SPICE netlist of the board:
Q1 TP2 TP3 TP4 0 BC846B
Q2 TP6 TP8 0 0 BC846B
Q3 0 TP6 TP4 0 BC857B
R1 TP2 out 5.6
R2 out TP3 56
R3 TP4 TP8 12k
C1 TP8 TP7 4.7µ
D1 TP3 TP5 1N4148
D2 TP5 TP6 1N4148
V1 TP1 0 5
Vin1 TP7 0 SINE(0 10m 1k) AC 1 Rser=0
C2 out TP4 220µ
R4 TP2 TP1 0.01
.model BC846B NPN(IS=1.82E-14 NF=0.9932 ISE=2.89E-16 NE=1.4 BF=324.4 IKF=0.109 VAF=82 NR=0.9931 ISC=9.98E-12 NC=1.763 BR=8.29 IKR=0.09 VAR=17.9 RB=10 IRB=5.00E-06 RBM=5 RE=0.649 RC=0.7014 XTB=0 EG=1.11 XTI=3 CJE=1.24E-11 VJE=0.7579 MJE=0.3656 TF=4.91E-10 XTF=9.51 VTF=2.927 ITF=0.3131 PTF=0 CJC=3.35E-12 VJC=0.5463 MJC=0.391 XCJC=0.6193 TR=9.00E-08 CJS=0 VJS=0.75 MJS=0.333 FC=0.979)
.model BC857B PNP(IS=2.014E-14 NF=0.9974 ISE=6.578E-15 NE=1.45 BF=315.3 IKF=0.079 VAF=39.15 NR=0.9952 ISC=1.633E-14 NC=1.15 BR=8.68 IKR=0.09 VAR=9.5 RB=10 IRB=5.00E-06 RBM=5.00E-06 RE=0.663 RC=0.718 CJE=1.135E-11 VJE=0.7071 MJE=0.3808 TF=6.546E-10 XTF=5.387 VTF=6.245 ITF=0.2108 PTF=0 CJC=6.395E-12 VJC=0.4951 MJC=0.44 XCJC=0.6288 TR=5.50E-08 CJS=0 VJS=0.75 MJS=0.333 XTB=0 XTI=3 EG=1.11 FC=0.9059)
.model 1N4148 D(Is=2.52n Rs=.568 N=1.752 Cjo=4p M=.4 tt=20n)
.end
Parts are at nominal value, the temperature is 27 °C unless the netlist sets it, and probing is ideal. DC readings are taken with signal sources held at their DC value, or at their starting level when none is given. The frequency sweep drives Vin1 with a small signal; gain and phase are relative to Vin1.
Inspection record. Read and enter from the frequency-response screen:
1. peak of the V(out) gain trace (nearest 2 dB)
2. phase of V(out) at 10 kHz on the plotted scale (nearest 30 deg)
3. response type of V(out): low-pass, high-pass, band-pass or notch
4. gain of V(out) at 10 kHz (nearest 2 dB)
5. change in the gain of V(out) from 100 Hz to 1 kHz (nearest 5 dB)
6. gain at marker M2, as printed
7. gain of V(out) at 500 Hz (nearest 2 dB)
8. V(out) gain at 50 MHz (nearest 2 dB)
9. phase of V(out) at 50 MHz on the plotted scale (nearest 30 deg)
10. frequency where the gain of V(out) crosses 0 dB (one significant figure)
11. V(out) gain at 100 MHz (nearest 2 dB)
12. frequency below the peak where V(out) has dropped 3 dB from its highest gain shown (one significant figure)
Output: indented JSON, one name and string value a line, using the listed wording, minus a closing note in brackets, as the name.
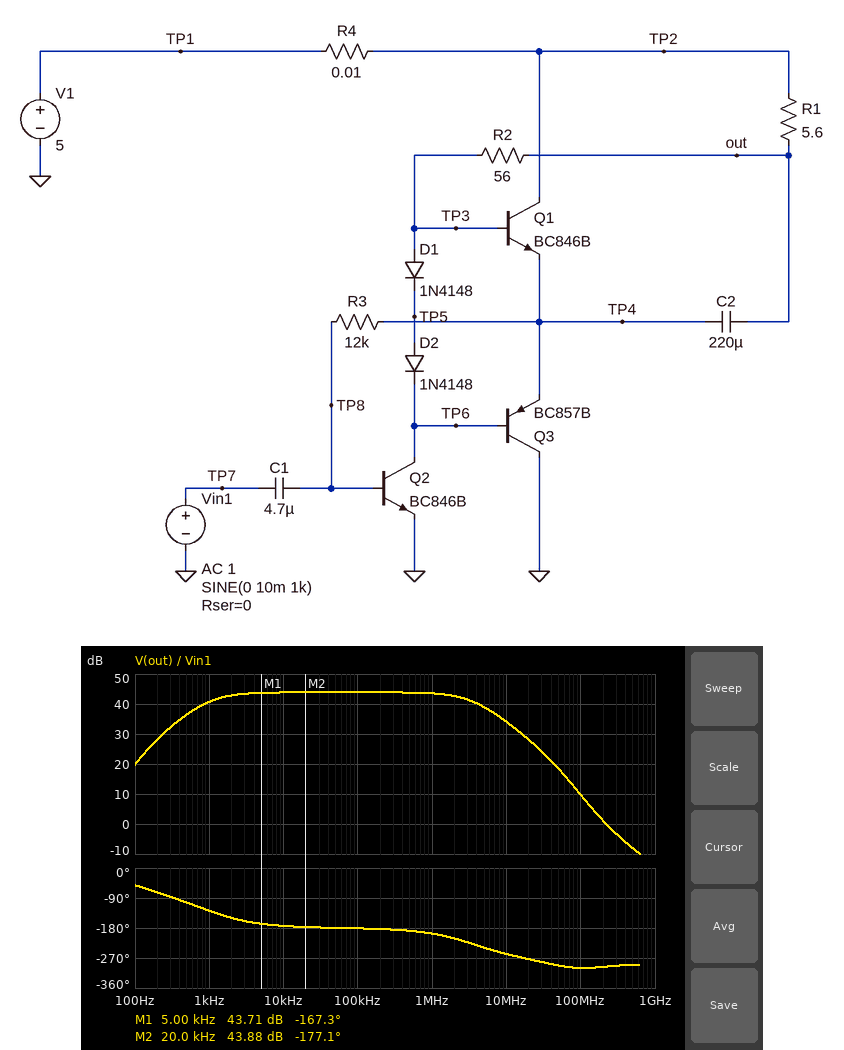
{
  "peak of the V(out) gain trace": "44 dB",
  "phase of V(out) at 10 kHz on the plotted scale": "-180 deg",
  "response type of V(out): low-pass, high-pass, band-pass or notch": "band-pass",
  "gain of V(out) at 10 kHz": "44 dB",
  "change in the gain of V(out) from 100 Hz to 1 kHz": "20 dB",
  "gain at marker M2, as printed": "43.88 dB",
  "gain of V(out) at 500 Hz": "36 dB",
  "V(out) gain at 50 MHz": "18 dB",
  "phase of V(out) at 50 MHz on the plotted scale": "-300 deg",
  "frequency where the gain of V(out) crosses 0 dB": "200 MHz",
  "V(out) gain at 100 MHz": "10 dB",
  "frequency below the peak where V(out) has dropped 3 dB from its highest gain shown": "1 kHz"
}
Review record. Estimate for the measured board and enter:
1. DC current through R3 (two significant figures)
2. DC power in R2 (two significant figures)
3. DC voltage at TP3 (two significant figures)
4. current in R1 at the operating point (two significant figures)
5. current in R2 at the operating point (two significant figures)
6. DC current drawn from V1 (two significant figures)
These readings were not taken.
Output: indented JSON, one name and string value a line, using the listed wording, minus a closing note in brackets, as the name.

{
  "DC current through R3": "130 µA",
  "DC power in R2": "55 mW",
  "DC voltage at TP3": "3.1 V",
  "current in R1 at the operating point": "31 mA",
  "current in R2 at the operating point": "31 mA",
  "DC current drawn from V1": "65 mA"
}
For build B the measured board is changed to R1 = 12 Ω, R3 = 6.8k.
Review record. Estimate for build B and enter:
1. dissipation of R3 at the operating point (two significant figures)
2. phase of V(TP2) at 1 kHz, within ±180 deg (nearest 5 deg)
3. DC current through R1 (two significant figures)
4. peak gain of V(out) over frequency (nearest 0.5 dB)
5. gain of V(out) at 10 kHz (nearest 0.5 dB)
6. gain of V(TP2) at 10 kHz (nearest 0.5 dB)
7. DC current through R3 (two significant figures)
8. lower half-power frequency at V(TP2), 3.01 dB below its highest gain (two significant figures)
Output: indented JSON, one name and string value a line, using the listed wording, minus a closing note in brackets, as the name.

{
  "dissipation of R3 at the operating point": "160 µW",
  "phase of V(TP2) at 1 kHz, within ±180 deg": "-110 deg",
  "DC current through R1": "36 mA",
  "peak gain of V(out) over frequency": "50.5 dB",
  "gain of V(out) at 10 kHz": "50.0 dB",
  "gain of V(TP2) at 10 kHz": "-17.0 dB",
  "DC current through R3": "150 µA",
  "lower half-power frequency at V(TP2), 3.01 dB below its highest gain": "2.3 kHz"
}
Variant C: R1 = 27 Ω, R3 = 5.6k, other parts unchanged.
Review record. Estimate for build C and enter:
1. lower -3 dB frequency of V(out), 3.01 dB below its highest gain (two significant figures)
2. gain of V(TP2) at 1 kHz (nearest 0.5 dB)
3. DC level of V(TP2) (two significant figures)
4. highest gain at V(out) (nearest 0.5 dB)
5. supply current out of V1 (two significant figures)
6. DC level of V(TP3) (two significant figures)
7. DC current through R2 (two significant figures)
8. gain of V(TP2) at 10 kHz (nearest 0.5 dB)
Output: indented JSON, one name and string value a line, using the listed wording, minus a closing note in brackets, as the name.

{
  "lower -3 dB frequency of V(out), 3.01 dB below its highest gain": "4.2 kHz",
  "gain of V(TP2) at 1 kHz": "-31.5 dB",
  "DC level of V(TP2)": "5.0 V",
  "highest gain at V(out)": "55.5 dB",
  "supply current out of V1": "68 mA",
  "DC level of V(TP3)": "2.3 V",
  "DC current through R2": "33 mA",
  "gain of V(TP2) at 10 kHz": "-19.5 dB"
}
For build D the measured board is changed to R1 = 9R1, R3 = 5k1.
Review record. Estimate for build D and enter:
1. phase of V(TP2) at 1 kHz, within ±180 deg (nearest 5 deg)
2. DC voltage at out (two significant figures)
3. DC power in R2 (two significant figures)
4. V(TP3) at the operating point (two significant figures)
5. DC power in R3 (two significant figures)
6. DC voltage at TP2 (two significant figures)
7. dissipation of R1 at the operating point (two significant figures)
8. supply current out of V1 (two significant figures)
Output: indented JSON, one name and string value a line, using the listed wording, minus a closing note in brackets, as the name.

{
  "phase of V(TP2) at 1 kHz, within ±180 deg": "-110 deg",
  "DC voltage at out": "4.6 V",
  "DC power in R2": "87 mW",
  "V(TP3) at the operating point": "2.4 V",
  "DC power in R3": "160 µW",
  "DC voltage at TP2": "5.0 V",
  "dissipation of R1 at the operating point": "14 mW",
  "supply current out of V1": "83 mA"
}
